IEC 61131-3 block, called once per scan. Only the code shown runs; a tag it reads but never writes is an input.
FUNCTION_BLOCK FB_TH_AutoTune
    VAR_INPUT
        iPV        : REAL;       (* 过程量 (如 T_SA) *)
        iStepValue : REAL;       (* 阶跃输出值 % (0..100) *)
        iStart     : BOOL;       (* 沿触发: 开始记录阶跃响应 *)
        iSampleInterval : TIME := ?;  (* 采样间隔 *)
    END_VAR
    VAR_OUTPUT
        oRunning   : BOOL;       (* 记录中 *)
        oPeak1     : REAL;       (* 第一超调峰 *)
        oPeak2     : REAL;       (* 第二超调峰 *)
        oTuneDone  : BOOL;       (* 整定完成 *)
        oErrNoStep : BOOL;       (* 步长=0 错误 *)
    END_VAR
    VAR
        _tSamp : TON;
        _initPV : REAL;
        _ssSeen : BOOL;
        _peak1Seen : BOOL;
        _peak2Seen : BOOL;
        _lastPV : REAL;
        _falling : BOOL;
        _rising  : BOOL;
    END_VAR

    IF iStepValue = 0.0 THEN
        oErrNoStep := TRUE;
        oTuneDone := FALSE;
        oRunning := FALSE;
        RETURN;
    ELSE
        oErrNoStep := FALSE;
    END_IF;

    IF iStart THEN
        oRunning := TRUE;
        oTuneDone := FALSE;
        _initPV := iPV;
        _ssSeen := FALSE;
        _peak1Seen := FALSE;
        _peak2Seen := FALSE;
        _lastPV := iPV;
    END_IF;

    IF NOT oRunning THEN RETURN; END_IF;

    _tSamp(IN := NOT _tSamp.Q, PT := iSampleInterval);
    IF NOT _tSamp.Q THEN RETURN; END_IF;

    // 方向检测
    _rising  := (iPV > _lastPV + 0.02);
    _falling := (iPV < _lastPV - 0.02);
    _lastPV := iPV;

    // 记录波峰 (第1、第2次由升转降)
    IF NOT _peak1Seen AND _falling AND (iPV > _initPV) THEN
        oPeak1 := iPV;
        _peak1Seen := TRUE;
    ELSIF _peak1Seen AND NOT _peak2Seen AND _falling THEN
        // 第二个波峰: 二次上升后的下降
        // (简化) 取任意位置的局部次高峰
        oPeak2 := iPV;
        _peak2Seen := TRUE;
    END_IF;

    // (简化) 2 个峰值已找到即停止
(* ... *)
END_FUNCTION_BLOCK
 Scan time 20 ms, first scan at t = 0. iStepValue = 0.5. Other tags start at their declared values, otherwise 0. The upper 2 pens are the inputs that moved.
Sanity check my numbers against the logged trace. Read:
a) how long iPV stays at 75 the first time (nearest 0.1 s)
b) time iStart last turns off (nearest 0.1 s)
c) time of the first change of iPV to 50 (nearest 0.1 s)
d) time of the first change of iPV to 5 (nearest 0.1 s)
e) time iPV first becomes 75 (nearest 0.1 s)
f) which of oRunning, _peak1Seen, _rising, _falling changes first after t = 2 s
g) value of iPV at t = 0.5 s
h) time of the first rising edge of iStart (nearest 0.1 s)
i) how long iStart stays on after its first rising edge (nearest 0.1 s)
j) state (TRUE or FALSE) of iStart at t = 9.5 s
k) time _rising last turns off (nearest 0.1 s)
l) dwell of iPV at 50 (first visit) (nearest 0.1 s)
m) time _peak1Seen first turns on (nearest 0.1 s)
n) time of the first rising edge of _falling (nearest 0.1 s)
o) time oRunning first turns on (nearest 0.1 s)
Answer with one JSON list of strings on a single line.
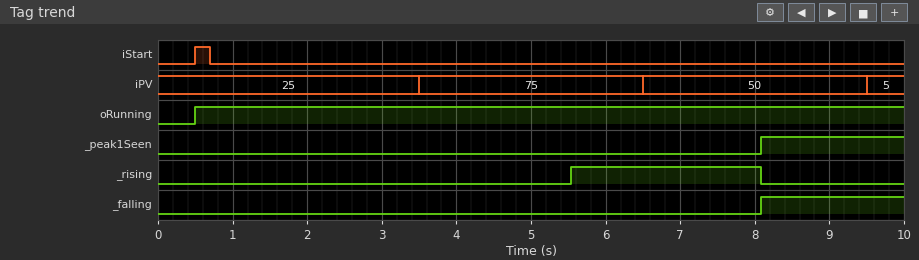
["3.0 s", "0.7 s", "6.5 s", "9.5 s", "3.5 s", "_rising", "25", "0.5 s", "0.2 s", "FALSE", "8.1 s", "3.0 s", "8.1 s", "8.1 s", "0.5 s"]
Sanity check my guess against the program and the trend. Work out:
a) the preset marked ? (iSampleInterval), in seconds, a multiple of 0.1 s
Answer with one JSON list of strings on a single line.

["2.5 s"]
